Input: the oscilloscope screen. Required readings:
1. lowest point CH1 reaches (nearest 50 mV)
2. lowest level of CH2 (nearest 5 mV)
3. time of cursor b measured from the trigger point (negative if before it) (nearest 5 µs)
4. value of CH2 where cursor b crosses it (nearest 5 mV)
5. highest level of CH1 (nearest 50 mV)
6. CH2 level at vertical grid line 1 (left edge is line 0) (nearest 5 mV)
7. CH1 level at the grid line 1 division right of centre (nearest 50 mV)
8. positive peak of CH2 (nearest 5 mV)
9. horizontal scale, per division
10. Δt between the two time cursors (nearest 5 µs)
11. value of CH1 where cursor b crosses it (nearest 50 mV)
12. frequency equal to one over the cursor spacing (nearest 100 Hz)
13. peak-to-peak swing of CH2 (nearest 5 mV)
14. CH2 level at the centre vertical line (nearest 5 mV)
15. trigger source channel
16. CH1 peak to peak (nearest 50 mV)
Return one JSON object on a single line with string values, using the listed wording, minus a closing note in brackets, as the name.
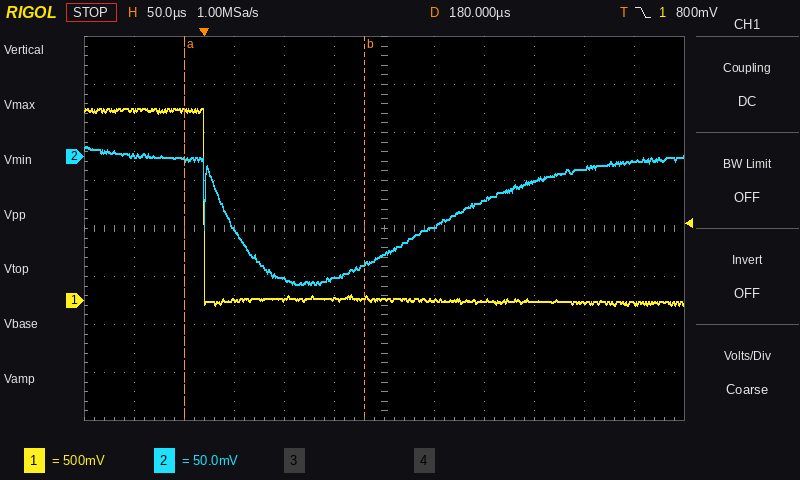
{"lowest point CH1 reaches": "-50 mV", "lowest level of CH2": "-135 mV", "time of cursor b measured from the trigger point (negative if before it)": "+160 µs", "value of CH2 where cursor b crosses it": "-110 mV", "highest level of CH1": "2.00 V", "CH2 level at vertical grid line 1 (left edge is line 0)": "0 mV", "CH1 level at the grid line 1 division right of centre": "0 mV", "positive peak of CH2": "10 mV", "horizontal scale, per division": "50 µs", "Δt between the two time cursors": "180 µs", "value of CH1 where cursor b crosses it": "50 mV", "frequency equal to one over the cursor spacing": "5.6 kHz", "peak-to-peak swing of CH2": "145 mV", "CH2 level at the centre vertical line": "-100 mV", "trigger source channel": "CH1", "CH1 peak to peak": "2.05 V"}
